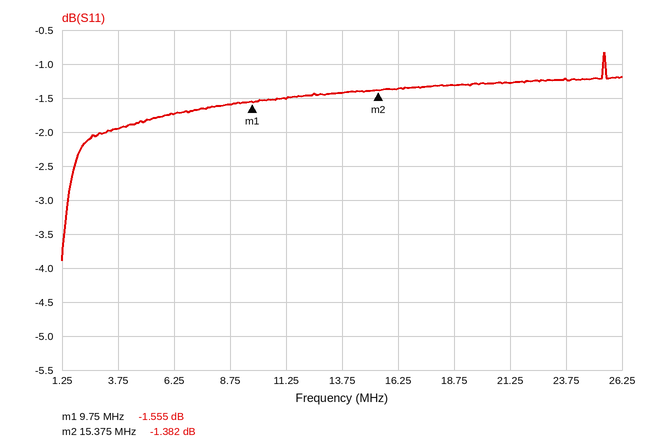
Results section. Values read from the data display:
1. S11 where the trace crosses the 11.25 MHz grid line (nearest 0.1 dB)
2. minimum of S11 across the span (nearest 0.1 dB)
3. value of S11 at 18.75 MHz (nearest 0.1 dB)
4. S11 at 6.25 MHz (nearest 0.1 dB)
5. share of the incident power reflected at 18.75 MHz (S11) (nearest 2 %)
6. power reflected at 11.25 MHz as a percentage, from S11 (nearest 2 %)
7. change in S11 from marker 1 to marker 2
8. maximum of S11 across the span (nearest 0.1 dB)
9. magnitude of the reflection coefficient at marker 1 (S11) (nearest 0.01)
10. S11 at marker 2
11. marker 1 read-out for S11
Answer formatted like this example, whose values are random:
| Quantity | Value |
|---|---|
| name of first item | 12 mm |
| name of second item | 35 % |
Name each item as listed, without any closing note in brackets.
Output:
| Quantity | Value |
|---|---|
| S11 where the trace crosses the 11.25 MHz grid line | -1.5 dB |
| minimum of S11 across the span | -3.9 dB |
| value of S11 at 18.75 MHz | -1.3 dB |
| S11 at 6.25 MHz | -1.7 dB |
| share of the incident power reflected at 18.75 MHz (S11) | 74 % |
| power reflected at 11.25 MHz as a percentage, from S11 | 70 % |
| change in S11 from marker 1 to marker 2 | 0.173 dB |
| maximum of S11 across the span | -0.8 dB |
| magnitude of the reflection coefficient at marker 1 (S11) | 0.84 |
| S11 at marker 2 | -1.382 dB |
| marker 1 read-out for S11 | -1.555 dB |
